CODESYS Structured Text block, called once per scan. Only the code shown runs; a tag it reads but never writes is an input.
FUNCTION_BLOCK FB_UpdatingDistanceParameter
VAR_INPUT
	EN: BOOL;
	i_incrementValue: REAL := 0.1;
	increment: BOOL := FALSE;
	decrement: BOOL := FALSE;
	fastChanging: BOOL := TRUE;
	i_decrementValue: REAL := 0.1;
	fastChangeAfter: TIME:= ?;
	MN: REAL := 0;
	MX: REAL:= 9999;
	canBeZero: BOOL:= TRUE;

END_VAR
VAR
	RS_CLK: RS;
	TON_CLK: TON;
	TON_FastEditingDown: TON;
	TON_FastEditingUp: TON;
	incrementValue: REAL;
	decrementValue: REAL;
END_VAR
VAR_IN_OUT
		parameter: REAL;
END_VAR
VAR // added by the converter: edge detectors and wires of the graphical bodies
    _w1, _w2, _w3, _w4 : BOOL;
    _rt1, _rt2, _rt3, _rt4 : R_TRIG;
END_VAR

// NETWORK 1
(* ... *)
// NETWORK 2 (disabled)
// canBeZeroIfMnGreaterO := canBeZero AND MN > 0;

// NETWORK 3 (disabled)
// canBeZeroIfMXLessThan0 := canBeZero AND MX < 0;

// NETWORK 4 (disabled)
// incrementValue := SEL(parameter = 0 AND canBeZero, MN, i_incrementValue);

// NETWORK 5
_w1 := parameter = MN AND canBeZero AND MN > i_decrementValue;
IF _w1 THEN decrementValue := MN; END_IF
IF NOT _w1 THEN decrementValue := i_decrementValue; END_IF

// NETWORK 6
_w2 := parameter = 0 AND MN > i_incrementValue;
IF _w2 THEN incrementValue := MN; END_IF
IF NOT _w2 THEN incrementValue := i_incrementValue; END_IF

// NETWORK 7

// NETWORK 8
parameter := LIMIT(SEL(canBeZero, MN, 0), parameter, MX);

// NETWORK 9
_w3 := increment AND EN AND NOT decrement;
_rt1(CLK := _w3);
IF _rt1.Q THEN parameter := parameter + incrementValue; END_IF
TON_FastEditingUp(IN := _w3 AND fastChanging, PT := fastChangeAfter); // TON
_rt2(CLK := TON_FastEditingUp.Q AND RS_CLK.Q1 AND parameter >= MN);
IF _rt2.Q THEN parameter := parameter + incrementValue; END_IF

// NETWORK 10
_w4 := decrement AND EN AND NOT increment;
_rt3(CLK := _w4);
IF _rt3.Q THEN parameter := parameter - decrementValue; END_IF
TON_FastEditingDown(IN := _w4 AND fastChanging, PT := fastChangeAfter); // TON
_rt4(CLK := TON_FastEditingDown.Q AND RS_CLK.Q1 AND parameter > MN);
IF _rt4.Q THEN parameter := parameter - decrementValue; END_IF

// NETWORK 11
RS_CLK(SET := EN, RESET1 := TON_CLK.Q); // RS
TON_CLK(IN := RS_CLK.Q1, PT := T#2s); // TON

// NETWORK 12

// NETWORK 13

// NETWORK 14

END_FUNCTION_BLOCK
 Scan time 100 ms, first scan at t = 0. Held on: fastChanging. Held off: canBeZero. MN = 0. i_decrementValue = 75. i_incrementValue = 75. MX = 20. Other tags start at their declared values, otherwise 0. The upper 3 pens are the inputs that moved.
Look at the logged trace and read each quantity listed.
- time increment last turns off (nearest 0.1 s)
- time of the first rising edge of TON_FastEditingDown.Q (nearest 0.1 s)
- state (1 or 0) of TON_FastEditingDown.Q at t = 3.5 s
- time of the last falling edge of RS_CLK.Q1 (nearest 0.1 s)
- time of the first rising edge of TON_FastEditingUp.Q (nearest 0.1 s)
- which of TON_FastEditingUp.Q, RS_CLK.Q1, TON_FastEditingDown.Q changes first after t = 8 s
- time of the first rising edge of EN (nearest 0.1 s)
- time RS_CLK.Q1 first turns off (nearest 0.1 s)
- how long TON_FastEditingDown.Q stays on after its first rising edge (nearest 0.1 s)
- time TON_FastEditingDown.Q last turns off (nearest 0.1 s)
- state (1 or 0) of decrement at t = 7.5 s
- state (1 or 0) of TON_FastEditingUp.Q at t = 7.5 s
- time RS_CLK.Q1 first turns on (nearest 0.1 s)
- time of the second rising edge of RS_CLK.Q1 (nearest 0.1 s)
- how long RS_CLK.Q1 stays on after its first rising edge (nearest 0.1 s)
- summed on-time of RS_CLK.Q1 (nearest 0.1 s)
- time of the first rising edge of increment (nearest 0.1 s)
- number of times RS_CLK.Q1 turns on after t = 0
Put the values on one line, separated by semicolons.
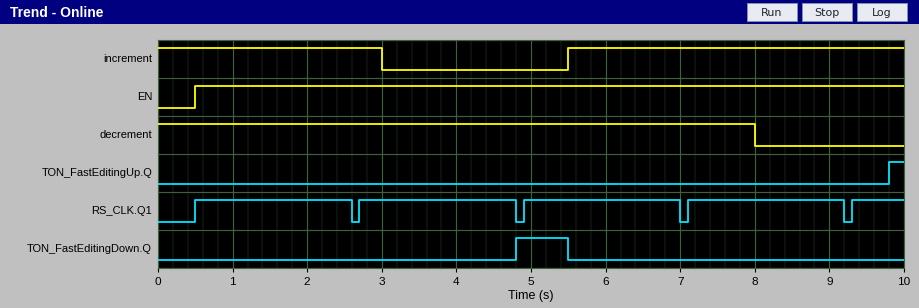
3.0 s; 4.8 s; 0; 9.2 s; 9.8 s; RS_CLK.Q1; 0.5 s; 2.6 s; 0.7 s; 5.5 s; 1; 0; 0.5 s; 2.7 s; 2.1 s; 9.1 s; 5.5 s; 5
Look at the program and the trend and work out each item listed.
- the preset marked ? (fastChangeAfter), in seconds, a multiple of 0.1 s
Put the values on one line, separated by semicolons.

1.8 s
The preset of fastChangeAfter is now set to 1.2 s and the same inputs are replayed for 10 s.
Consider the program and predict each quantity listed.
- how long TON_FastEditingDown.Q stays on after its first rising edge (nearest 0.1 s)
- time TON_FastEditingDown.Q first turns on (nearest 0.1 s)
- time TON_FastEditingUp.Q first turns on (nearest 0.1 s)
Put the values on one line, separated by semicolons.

1.3 s; 4.2 s; 9.2 s
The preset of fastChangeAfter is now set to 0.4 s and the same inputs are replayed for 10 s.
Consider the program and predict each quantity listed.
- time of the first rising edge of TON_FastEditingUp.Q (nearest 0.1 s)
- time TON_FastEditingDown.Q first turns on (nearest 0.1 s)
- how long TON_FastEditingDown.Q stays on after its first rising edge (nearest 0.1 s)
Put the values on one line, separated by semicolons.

8.4 s; 3.4 s; 2.1 s
